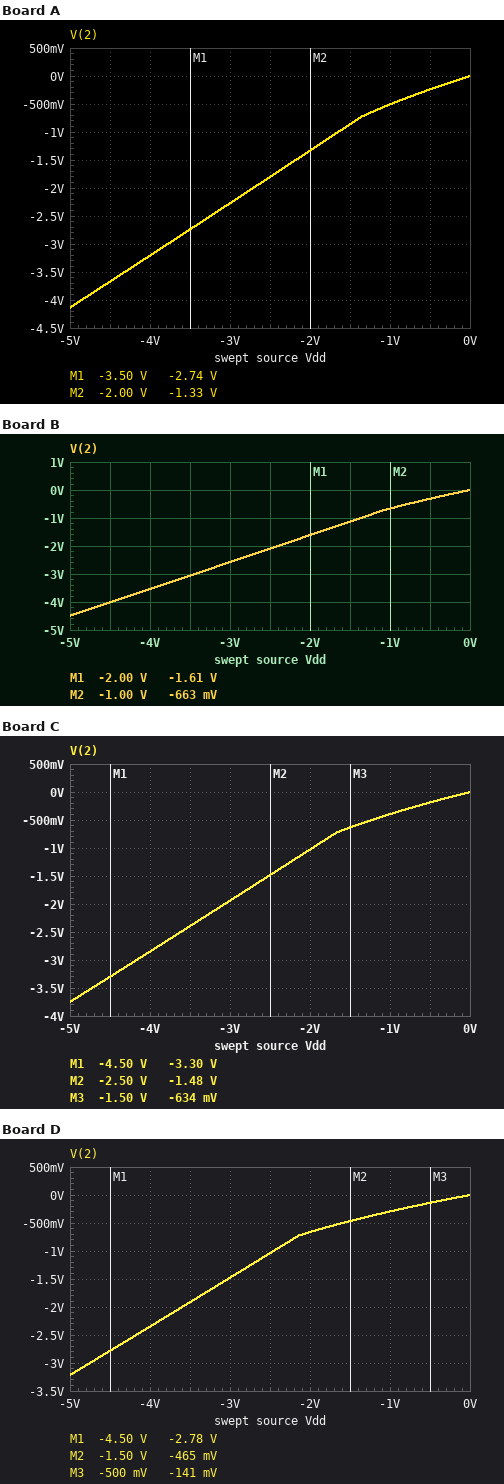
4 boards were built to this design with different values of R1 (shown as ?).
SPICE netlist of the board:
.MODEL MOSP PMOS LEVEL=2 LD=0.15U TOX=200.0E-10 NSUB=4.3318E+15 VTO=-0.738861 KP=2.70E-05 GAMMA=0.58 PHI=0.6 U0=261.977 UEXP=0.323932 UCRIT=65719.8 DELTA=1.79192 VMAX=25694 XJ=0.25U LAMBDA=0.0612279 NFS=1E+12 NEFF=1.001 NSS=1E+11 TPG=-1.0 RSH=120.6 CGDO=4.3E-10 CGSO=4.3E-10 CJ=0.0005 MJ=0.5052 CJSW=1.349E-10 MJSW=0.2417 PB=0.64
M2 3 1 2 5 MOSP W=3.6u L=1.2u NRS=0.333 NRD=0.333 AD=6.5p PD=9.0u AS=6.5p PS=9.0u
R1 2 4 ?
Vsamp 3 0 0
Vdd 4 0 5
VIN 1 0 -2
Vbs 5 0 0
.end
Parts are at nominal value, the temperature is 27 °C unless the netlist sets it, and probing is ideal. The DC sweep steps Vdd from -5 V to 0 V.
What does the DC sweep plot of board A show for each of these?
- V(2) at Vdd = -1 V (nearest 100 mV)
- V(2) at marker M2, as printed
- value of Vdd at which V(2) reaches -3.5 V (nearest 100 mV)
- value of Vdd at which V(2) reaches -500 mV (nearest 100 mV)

-500 mV
-1.33 V
-4.3 V
-1.0 V
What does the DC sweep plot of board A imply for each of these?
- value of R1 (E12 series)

12 kΩ
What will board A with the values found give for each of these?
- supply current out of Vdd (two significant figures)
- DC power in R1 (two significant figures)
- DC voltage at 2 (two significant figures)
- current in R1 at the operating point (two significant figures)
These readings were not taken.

360 µA
1.6 mW
640 mV
360 µA
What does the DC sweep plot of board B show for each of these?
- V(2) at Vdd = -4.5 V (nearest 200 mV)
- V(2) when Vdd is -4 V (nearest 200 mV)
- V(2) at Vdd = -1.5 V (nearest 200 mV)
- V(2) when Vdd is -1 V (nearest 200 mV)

-4.0 V
-3.6 V
-1.2 V
-600 mV
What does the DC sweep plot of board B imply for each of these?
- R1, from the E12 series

6.8 kΩ
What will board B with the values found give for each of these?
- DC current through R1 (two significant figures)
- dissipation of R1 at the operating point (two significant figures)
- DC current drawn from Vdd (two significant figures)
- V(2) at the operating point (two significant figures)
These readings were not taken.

640 µA
2.8 mW
640 µA
670 mV
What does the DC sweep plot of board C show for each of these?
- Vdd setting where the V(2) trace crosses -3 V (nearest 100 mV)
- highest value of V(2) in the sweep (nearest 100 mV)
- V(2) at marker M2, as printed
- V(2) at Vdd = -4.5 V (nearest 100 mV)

-4.2 V
0 V
-1.48 V
-3.3 V
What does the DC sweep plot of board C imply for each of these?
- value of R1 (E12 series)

18 kΩ
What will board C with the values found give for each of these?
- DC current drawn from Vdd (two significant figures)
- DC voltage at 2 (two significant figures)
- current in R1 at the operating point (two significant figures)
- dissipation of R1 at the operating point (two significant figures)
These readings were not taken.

240 µA
620 mV
240 µA
1.1 mW
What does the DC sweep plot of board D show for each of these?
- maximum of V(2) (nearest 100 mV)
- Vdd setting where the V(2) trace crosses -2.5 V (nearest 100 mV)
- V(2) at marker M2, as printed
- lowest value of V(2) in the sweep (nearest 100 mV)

0 V
-4.2 V
-465 mV
-3.2 V
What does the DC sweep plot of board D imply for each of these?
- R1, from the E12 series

27 kΩ
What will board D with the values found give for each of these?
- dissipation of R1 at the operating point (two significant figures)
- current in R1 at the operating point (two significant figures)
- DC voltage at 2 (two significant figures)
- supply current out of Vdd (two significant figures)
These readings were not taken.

720 µW
160 µA
600 mV
160 µA
